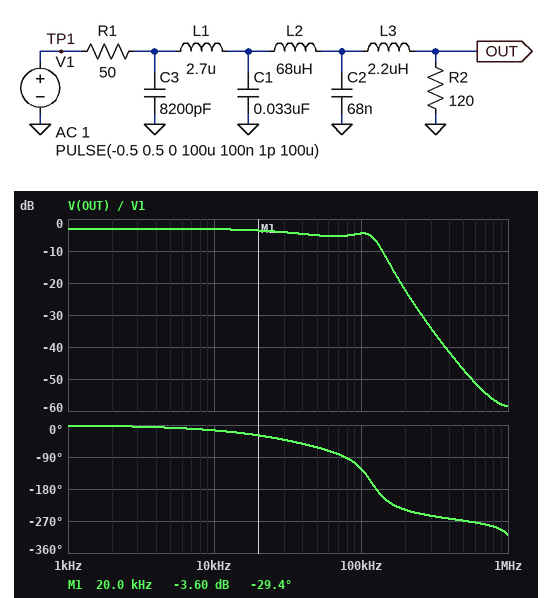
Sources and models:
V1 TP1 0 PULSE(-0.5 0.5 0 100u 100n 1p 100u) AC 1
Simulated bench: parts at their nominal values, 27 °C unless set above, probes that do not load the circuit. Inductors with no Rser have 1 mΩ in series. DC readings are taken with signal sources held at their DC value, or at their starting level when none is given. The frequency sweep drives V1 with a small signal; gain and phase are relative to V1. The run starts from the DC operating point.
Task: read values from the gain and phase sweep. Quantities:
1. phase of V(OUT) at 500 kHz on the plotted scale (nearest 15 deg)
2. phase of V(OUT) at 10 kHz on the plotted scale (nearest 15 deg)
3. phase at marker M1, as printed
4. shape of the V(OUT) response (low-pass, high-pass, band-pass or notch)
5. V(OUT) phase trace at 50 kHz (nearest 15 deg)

-270 deg
-15 deg
-29.4 deg
low-pass
-60 deg
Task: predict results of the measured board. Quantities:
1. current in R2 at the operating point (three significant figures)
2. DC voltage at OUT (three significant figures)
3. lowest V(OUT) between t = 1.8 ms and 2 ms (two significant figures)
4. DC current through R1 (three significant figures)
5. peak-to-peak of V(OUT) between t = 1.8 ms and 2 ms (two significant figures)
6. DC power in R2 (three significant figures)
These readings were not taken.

2.94 mA
-353 mV
-310 mV
2.94 mA
640 mV
1.04 mW
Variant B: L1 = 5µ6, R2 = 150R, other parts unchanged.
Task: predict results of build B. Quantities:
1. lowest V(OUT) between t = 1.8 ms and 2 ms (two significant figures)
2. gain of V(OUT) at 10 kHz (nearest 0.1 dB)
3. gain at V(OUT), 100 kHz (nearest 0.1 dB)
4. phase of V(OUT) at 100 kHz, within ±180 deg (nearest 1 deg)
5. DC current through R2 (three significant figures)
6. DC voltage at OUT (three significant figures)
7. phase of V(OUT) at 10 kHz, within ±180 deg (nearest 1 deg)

-320 mV
-2.7 dB
-4.3 dB
-126 deg
2.50 mA
-375 mV
-16 deg
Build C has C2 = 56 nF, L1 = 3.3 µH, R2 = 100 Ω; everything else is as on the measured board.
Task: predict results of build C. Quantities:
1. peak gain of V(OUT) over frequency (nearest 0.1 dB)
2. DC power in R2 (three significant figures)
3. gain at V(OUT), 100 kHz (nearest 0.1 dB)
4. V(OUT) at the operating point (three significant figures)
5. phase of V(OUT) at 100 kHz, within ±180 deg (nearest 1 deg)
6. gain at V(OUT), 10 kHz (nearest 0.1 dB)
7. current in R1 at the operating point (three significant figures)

-3.5 dB
1.11 mW
-4.3 dB
-333 mV
-112 deg
-3.6 dB
3.33 mA
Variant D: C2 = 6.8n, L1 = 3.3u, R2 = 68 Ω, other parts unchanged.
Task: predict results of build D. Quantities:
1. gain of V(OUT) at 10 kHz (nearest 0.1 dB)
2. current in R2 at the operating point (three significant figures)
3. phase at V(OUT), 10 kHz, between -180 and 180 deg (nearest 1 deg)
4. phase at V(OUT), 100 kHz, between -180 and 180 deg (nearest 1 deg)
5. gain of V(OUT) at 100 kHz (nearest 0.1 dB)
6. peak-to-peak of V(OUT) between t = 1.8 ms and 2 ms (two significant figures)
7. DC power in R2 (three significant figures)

-4.8 dB
4.24 mA
-7 deg
-71 deg
-6.1 dB
550 mV
1.22 mW
